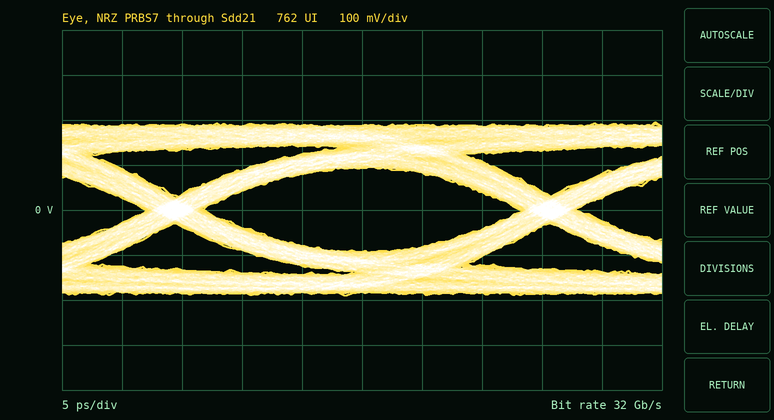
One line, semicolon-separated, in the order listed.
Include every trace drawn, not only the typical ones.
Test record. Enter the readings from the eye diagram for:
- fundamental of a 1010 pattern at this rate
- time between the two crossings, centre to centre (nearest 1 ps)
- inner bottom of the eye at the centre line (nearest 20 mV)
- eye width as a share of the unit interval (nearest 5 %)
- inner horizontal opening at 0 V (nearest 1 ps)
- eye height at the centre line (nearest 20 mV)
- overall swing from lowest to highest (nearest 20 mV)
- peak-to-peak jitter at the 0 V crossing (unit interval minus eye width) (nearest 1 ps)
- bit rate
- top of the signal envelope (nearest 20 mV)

16 GHz; 31 ps; -100 mV; 85 %; 26 ps; 180 mV; 380 mV; 5 ps; 32 Gb/s; 200 mV
